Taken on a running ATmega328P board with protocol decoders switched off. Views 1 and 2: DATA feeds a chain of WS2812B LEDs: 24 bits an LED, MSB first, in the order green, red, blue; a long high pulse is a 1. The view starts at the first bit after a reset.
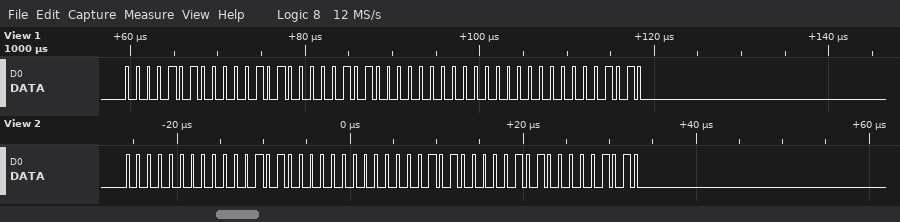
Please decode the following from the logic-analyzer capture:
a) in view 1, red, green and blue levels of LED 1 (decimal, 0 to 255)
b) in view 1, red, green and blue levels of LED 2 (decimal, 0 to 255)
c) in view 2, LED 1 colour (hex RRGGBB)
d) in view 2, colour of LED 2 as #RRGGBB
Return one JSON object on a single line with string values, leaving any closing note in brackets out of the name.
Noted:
{"in view 1, red, green and blue levels of LED 1": "10, 10, 10", "in view 1, red, green and blue levels of LED 2": "0, 0, 10", "in view 2, LED 1 colour": "#0A0000", "in view 2, colour of LED 2 as #RRGGBB": "#0A0A0A"}
